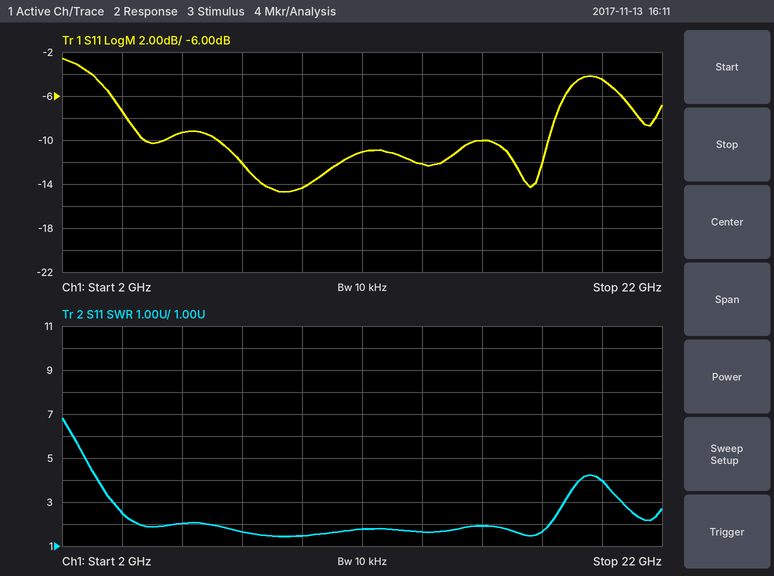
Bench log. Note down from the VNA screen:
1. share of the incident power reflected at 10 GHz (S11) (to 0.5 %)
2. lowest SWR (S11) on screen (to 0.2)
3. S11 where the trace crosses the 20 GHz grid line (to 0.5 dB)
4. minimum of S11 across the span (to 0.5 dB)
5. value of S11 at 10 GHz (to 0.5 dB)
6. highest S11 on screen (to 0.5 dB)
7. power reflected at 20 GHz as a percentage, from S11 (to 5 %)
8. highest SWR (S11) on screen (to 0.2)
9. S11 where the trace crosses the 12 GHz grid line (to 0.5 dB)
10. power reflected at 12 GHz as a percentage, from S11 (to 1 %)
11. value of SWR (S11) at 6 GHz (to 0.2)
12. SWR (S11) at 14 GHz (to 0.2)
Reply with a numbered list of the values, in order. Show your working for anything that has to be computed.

1. 10^(-14.5/10) ≈ 3.5 %
2. 1.4
3. -4.5 dB
4. -14.5 dB
5. -14.5 dB
6. -2.5 dB
7. 10^(-4.5/10) ≈ 35 %
8. 6.8
9. -11.0 dB
10. 10^(-11/10) ≈ 8 %
11. 2.0
12. 1.6
